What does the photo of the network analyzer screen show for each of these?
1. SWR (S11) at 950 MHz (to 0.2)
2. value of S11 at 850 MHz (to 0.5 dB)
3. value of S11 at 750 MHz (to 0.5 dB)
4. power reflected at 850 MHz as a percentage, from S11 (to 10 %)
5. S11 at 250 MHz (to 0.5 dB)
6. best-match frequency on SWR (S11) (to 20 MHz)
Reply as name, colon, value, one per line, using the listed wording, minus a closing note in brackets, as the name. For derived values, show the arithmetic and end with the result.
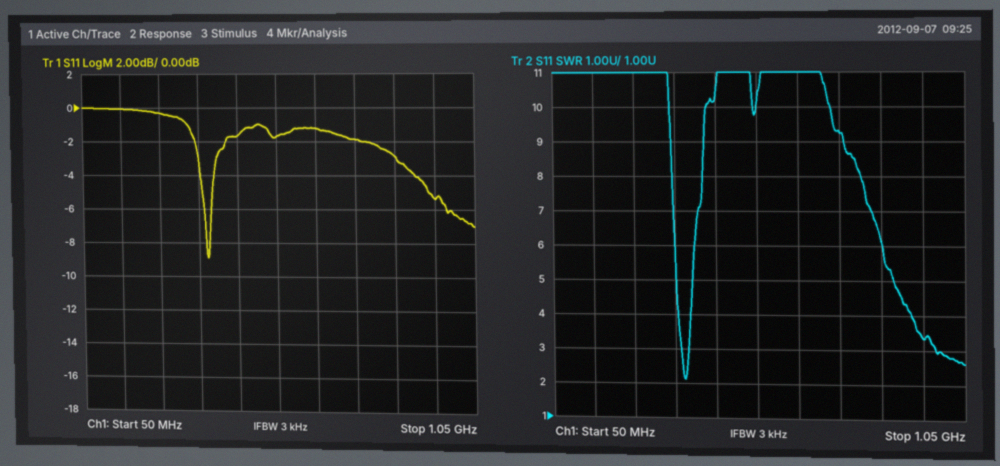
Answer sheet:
SWR (S11) at 950 MHz: 3.4
value of S11 at 850 MHz: -3.0 dB
value of S11 at 750 MHz: -2.0 dB
power reflected at 850 MHz as a percentage, from S11: 10^(-3/10) ≈ 50 %
S11 at 250 MHz: -0.5 dB
best-match frequency on SWR (S11): 380 MHz
